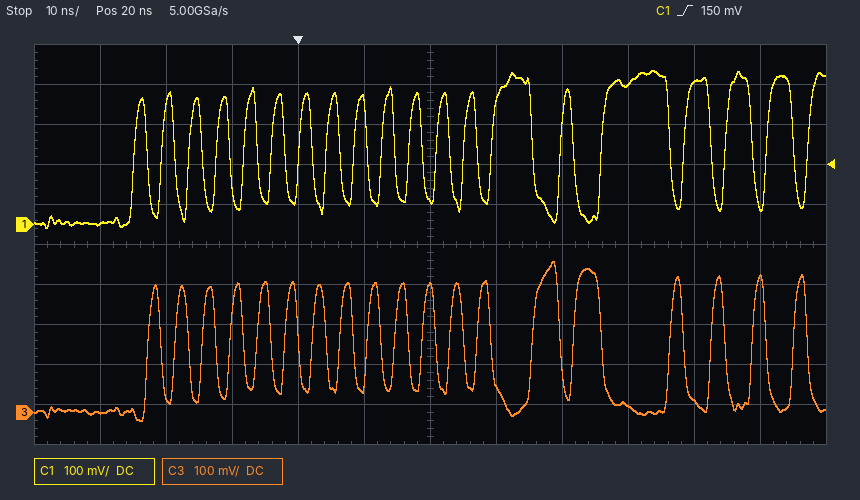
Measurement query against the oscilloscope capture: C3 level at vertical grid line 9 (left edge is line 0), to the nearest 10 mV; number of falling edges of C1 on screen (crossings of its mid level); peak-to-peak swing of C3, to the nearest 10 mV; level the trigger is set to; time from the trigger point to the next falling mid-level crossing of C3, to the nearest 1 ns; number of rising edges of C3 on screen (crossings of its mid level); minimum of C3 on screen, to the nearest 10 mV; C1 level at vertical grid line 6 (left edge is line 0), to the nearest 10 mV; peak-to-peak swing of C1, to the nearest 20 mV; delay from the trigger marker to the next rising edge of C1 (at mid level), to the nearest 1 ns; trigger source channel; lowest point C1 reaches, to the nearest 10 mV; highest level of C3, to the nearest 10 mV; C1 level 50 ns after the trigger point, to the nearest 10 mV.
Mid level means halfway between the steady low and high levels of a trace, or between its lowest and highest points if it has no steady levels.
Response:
20 mV
19
400 mV
150 mV
4 ns
19
-20 mV
60 mV
400 mV
4 ns
C1
-10 mV
380 mV
350 mV
